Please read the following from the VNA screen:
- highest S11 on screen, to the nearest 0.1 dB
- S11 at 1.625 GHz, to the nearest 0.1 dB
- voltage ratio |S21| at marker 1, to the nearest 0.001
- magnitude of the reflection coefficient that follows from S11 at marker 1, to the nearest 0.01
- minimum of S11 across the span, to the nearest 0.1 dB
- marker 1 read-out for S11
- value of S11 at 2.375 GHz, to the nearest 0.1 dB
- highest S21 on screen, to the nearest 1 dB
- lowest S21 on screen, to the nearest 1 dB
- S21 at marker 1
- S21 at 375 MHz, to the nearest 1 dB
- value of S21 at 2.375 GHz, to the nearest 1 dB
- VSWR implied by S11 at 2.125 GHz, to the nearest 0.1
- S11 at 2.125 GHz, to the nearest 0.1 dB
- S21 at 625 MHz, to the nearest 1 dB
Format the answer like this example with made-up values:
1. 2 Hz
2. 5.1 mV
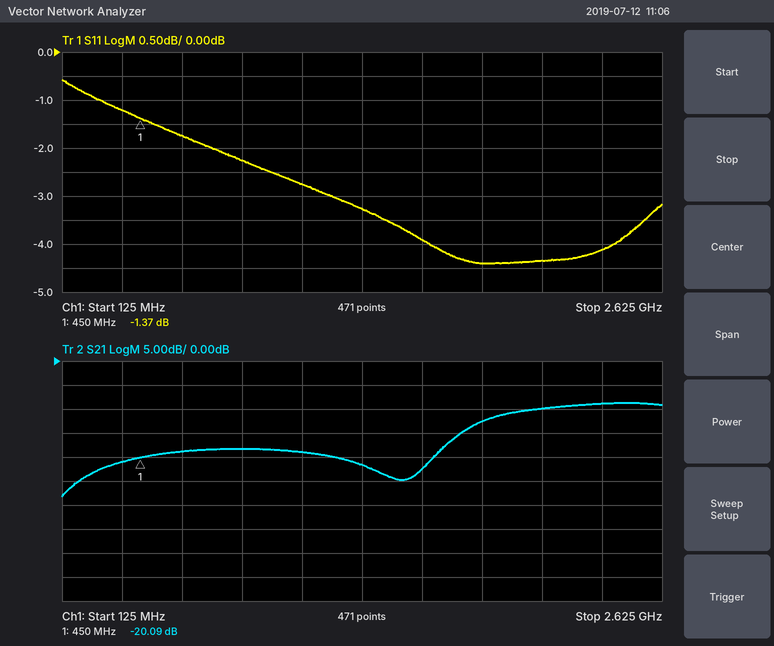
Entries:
1. -0.6 dB
2. -3.9 dB
3. 0.099
4. 0.85
5. -4.4 dB
6. -1.37 dB
7. -4.1 dB
8. -9 dB
9. -28 dB
10. -20.09 dB
11. -21 dB
12. -9 dB
13. 4.1
14. -4.3 dB
15. -19 dB
